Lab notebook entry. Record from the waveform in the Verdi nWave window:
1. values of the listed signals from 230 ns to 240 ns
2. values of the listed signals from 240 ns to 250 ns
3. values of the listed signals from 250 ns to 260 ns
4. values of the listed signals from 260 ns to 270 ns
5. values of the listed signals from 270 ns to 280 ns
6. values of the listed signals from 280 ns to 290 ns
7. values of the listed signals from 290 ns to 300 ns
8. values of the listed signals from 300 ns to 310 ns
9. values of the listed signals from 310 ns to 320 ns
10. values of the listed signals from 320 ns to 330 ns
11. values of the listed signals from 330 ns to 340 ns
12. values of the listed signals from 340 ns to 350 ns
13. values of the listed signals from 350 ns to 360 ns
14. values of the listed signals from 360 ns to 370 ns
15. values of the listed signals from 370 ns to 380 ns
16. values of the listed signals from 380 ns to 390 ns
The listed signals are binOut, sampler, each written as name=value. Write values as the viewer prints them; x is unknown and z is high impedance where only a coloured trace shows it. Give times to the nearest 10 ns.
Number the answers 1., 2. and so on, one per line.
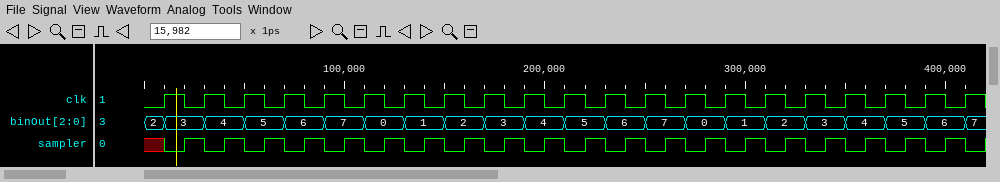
1. binOut=6, sampler=0
2. binOut=6, sampler=1
3. binOut=7, sampler=0
4. binOut=7, sampler=1
5. binOut=0, sampler=0
6. binOut=0, sampler=1
7. binOut=1, sampler=0
8. binOut=1, sampler=1
9. binOut=2, sampler=0
10. binOut=2, sampler=1
11. binOut=3, sampler=0
12. binOut=3, sampler=1
13. binOut=4, sampler=0
14. binOut=4, sampler=1
15. binOut=5, sampler=0
16. binOut=5, sampler=1
